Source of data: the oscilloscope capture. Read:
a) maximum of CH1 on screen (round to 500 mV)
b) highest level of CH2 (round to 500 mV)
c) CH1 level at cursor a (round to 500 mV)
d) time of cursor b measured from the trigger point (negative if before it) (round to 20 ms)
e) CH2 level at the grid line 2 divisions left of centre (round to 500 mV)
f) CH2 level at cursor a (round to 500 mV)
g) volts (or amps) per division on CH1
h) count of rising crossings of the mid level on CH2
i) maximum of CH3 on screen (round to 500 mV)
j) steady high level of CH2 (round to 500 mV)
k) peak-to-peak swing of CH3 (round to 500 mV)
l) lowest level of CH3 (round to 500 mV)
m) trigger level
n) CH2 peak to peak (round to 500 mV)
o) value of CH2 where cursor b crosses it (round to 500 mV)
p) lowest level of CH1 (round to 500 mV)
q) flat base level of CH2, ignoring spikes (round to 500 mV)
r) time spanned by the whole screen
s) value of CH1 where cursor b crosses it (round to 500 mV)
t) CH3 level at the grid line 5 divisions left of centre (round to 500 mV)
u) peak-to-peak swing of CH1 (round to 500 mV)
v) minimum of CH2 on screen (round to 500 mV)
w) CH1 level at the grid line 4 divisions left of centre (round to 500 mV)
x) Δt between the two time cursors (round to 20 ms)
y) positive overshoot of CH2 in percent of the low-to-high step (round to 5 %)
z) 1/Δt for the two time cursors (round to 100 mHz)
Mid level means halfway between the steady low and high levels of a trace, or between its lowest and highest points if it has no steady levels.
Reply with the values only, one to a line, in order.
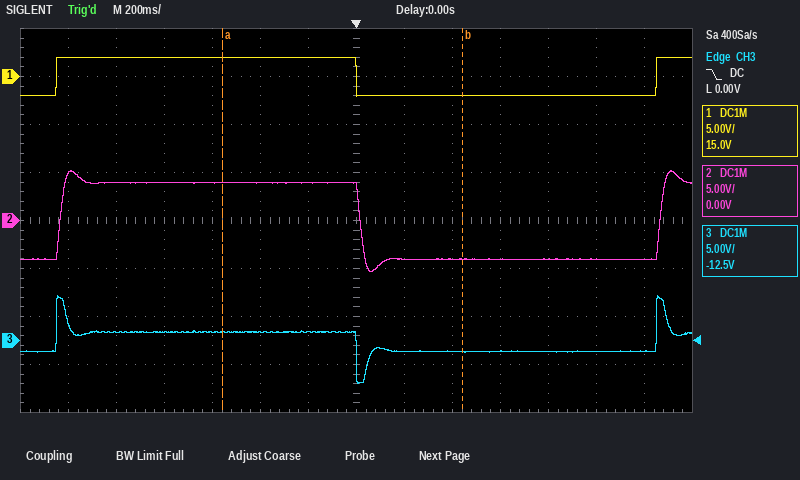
2.0 V
5.0 V
2.0 V
+440 ms
4.0 V
4.0 V
5 V
2
4.5 V
4.0 V
9.0 V
-4.5 V
0.00 V
10.5 V
-4.0 V
-2.0 V
-4.0 V
2.8 s
-2.0 V
1.0 V
4.0 V
-5.5 V
2.0 V
1.00 s
15 %
1.0 Hz
